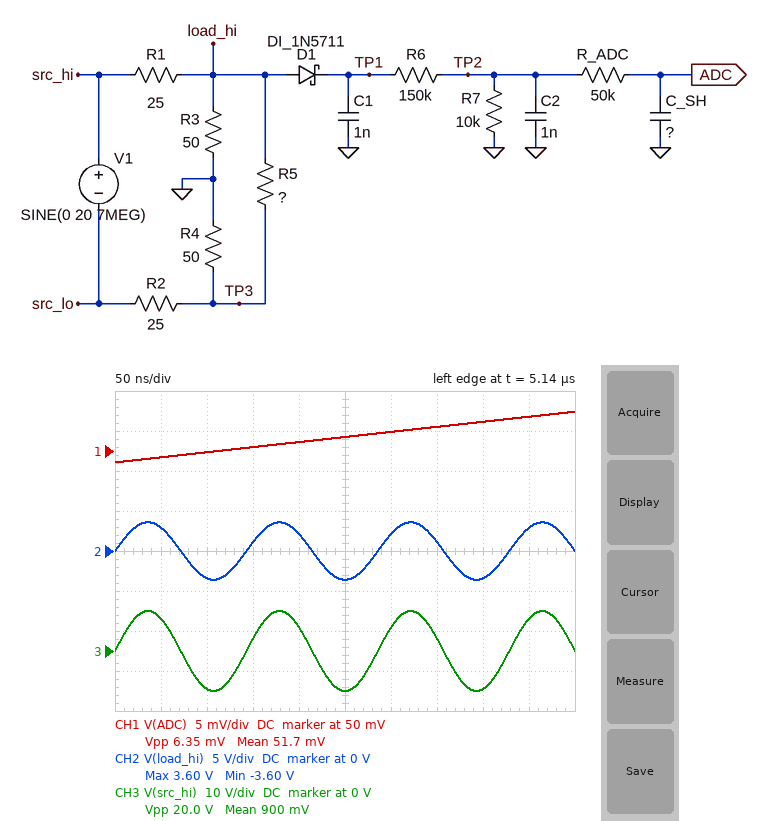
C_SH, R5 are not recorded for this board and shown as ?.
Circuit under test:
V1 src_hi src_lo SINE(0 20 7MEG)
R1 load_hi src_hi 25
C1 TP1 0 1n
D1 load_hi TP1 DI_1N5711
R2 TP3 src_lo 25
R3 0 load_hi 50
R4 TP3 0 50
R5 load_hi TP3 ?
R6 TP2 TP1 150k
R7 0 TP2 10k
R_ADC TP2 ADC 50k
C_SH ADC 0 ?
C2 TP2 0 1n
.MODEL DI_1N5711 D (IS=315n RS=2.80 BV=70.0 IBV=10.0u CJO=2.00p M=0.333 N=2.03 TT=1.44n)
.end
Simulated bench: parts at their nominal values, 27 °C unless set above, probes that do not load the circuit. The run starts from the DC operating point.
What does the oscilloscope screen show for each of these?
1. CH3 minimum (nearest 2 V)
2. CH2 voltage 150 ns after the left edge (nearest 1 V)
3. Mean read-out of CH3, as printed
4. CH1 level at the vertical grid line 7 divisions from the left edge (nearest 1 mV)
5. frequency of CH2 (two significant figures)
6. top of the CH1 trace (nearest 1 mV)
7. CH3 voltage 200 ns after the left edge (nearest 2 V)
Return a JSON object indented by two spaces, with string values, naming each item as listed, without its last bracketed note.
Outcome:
{
  "CH3 minimum": "-10 V",
  "CH2 voltage 150 ns after the left edge": "1 V",
  "Mean read-out of CH3, as printed": "900 mV",
  "CH1 level at the vertical grid line 7 divisions from the left edge": "53 mV",
  "frequency of CH2": "7.0 MHz",
  "top of the CH1 trace": "55 mV",
  "CH3 voltage 200 ns after the left edge": "6 V"
}
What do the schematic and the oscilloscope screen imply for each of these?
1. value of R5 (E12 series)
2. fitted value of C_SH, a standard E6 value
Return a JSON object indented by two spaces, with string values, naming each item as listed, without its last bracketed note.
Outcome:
{
  "value of R5": "39 Ω",
  "fitted value of C_SH, a standard E6 value": "47 pF"
}
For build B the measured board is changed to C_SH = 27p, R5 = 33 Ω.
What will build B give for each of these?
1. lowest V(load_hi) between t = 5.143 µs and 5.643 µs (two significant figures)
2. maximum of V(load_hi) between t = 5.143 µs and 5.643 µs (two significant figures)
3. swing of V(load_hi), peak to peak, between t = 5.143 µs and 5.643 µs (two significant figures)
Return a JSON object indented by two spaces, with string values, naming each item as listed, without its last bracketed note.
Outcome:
{
  "lowest V(load_hi) between t = 5.143 µs and 5.643 µs": "-3.3 V",
  "maximum of V(load_hi) between t = 5.143 µs and 5.643 µs": "3.3 V",
  "swing of V(load_hi), peak to peak, between t = 5.143 µs and 5.643 µs": "6.6 V"
}
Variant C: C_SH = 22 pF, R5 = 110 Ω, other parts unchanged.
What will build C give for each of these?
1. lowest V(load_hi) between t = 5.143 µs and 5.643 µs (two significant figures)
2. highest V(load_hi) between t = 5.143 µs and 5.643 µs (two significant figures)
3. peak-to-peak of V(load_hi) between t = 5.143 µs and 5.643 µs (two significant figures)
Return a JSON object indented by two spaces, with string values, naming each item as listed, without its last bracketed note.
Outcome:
{
  "lowest V(load_hi) between t = 5.143 µs and 5.643 µs": "-5.1 V",
  "highest V(load_hi) between t = 5.143 µs and 5.643 µs": "5.1 V",
  "peak-to-peak of V(load_hi) between t = 5.143 µs and 5.643 µs": "10 V"
}
